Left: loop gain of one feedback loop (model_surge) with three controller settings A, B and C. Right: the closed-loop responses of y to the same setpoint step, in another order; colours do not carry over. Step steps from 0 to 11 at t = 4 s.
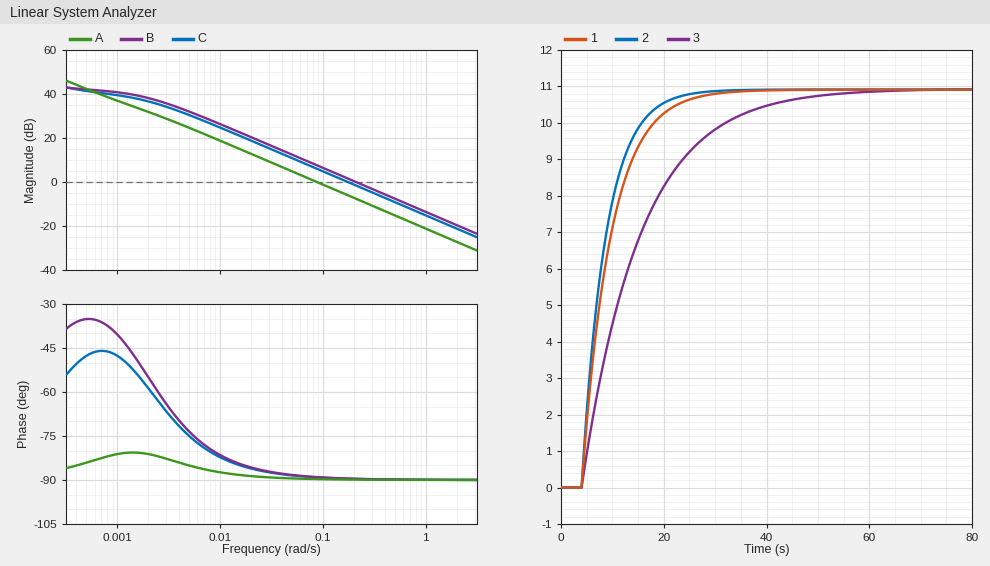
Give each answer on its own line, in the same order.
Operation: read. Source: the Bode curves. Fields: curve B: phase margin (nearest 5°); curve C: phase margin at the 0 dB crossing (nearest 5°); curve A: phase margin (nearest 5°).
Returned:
90°
90°
90°
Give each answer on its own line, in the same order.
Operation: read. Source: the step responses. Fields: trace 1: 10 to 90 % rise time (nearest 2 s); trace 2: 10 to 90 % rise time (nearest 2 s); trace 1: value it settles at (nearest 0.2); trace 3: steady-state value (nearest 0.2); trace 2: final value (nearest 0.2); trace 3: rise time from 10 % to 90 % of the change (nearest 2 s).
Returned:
12 s
10 s
11.0
11.0
11.0
26 s
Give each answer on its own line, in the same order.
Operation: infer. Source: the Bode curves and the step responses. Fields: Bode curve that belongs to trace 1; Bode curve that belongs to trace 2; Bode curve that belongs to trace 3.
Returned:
C
B
A
